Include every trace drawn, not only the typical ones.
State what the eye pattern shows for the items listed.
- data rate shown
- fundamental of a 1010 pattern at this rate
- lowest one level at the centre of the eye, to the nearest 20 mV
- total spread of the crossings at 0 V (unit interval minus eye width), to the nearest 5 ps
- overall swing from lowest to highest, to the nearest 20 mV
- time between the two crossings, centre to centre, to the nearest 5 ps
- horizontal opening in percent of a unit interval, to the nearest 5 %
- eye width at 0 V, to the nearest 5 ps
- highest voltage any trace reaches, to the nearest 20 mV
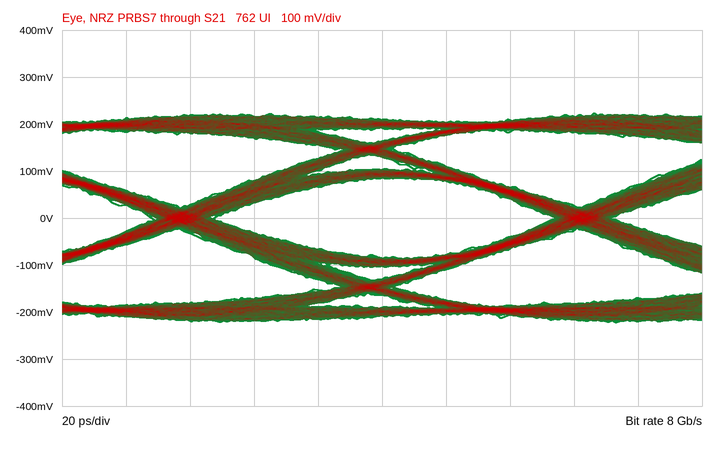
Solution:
8 Gb/s
4 GHz
80 mV
20 ps
440 mV
125 ps
85 %
105 ps
220 mV
